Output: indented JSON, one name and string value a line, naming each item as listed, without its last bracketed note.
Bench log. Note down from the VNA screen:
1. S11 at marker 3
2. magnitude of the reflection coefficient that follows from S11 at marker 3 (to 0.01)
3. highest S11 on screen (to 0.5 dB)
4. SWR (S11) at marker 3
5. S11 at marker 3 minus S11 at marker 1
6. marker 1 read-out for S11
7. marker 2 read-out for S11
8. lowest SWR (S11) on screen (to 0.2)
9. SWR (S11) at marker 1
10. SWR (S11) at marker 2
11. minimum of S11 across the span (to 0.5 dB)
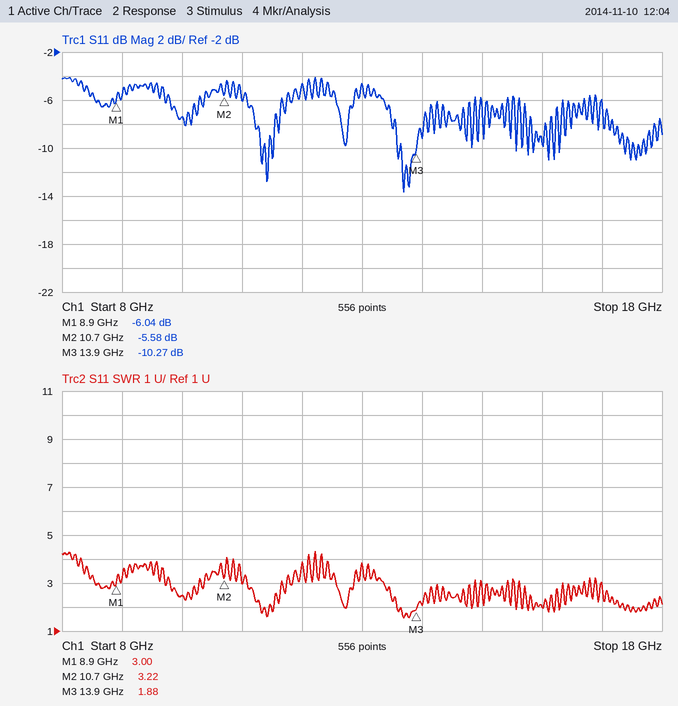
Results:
{
  "S11 at marker 3": "-10.27 dB",
  "magnitude of the reflection coefficient that follows from S11 at marker 3": "0.31",
  "highest S11 on screen": "-4.0 dB",
  "SWR (S11) at marker 3": "1.88",
  "S11 at marker 3 minus S11 at marker 1": "-4.23 dB",
  "marker 1 read-out for S11": "-6.04 dB",
  "marker 2 read-out for S11": "-5.58 dB",
  "lowest SWR (S11) on screen": "1.6",
  "SWR (S11) at marker 1": "3.00",
  "SWR (S11) at marker 2": "3.22",
  "minimum of S11 across the span": "-13.5 dB"
}
